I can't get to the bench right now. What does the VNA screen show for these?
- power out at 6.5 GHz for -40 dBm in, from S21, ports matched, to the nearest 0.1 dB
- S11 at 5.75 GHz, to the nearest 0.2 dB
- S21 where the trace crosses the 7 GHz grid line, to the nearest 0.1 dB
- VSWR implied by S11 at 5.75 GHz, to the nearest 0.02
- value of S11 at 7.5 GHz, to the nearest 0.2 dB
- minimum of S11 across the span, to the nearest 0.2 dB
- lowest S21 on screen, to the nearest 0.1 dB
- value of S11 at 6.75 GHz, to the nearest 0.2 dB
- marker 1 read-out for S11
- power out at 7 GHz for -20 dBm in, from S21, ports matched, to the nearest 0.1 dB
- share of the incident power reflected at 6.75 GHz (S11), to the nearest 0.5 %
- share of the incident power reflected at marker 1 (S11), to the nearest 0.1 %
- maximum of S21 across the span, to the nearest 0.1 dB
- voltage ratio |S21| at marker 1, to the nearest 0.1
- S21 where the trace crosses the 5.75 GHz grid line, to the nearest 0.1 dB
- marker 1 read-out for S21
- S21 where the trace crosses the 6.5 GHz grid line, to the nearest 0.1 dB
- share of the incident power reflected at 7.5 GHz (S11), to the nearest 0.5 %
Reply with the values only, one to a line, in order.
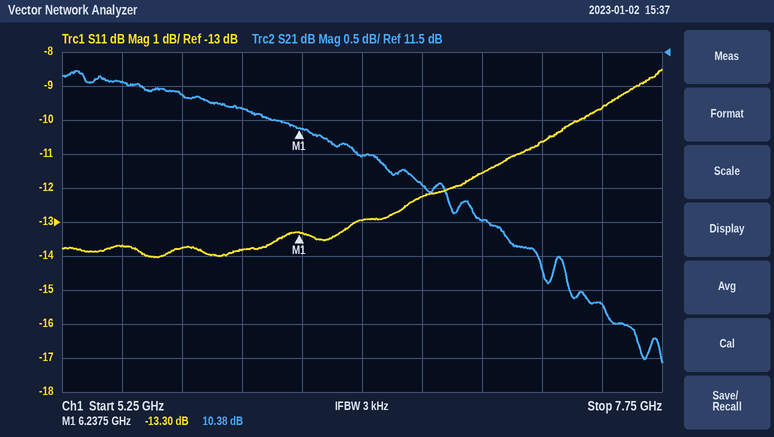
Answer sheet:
-30.0 dBm
-13.8 dB
9.0 dB
1.52
-9.6 dB
-14.0 dB
6.9 dB
-12.2 dB
-13.30 dB
-11.0 dBm
6.0 %
4.7 %
11.2 dB
3.3
10.9 dB
10.38 dB
10.0 dB
11.0 %
